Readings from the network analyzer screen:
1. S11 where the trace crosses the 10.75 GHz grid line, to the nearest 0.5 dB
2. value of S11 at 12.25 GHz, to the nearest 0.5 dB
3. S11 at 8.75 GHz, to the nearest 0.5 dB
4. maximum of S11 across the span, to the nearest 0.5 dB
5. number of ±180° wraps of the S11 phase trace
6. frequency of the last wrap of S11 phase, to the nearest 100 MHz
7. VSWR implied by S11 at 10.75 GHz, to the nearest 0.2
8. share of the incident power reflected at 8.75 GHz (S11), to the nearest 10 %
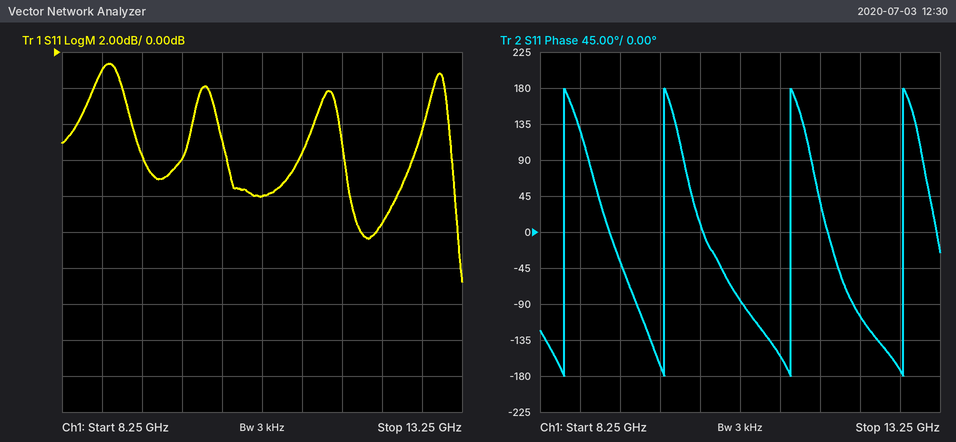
-8.0 dB
-9.5 dB
-1.0 dB
-0.5 dB
4
12.8 GHz
2.4
80 %
